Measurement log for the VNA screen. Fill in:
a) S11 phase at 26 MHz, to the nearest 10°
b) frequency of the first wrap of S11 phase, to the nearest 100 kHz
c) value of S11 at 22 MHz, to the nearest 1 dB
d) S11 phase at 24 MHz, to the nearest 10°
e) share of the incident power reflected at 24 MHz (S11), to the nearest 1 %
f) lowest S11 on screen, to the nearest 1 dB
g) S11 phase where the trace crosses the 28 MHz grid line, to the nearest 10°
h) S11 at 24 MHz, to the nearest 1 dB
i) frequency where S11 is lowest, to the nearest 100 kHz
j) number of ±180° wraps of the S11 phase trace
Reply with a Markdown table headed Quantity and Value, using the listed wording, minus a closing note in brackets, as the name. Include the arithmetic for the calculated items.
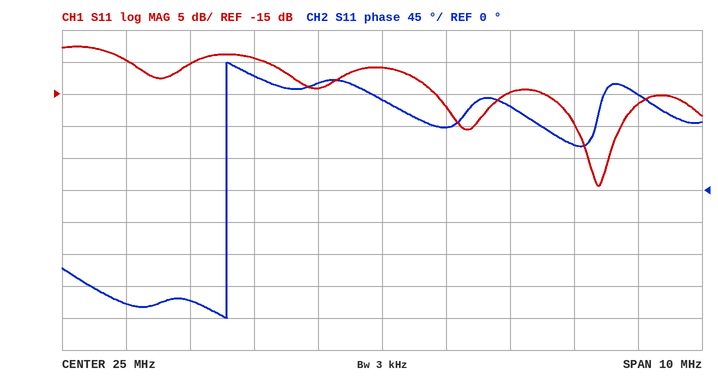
| Quantity | Value |
|---|---|
| S11 phase at 26 MHz, to the nearest 10° | 90° |
| frequency of the first wrap of S11 phase, to the nearest 100 kHz | 22.6 MHz |
| value of S11 at 22 MHz, to the nearest 1 dB | -10 dB |
| S11 phase at 24 MHz, to the nearest 10° | 150° |
| share of the incident power reflected at 24 MHz (S11), to the nearest 1 % | 10^(-14/10) ≈ 4 % |
| lowest S11 on screen, to the nearest 1 dB | -29 dB |
| S11 phase where the trace crosses the 28 MHz grid line, to the nearest 10° | 60° |
| S11 at 24 MHz, to the nearest 1 dB | -14 dB |
| frequency where S11 is lowest, to the nearest 100 kHz | 28.4 MHz |
| number of ±180° wraps of the S11 phase trace | 1 |
